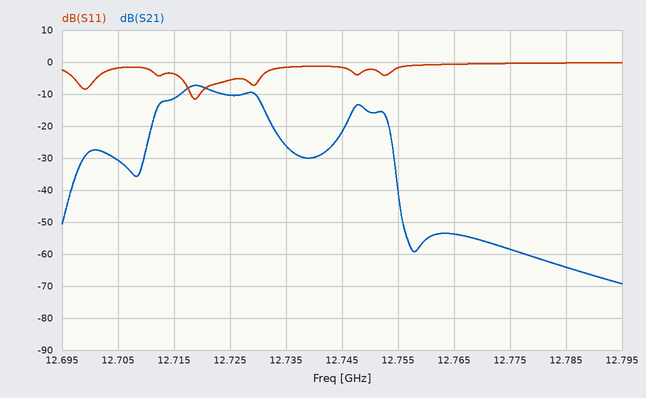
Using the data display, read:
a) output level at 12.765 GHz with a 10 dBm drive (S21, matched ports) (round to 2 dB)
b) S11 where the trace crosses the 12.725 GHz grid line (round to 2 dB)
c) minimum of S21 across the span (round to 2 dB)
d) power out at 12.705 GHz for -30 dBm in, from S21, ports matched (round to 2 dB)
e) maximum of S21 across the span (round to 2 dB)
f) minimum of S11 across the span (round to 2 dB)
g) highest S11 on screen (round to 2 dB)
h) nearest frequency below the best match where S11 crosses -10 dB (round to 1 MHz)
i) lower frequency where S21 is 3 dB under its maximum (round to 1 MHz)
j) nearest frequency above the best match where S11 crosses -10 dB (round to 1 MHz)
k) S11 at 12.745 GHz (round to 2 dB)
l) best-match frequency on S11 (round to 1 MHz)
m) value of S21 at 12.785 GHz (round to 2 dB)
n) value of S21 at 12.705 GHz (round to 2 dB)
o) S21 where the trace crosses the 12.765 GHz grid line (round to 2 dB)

-44 dBm
-6 dB
-70 dB
-60 dBm
-8 dB
-12 dB
0 dB
12.718 GHz
12.716 GHz
12.720 GHz
-2 dB
12.719 GHz
-64 dB
-30 dB
-54 dB
